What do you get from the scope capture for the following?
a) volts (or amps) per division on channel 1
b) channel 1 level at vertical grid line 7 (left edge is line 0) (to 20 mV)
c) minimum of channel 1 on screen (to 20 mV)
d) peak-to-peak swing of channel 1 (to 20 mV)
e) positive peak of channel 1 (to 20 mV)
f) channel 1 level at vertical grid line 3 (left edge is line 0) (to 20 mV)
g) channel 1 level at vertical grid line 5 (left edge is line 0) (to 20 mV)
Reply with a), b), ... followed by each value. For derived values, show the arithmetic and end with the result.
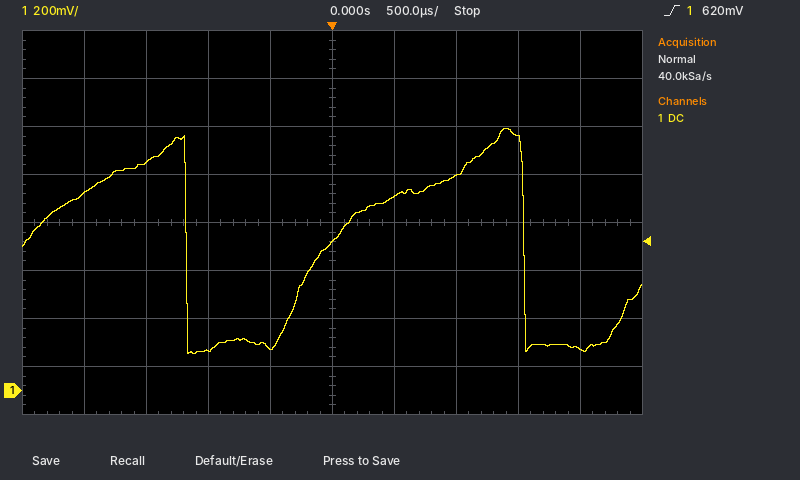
a) 200 mV
b) 900 mV
c) 160 mV
d) 1.10 V − (160 mV) = 940 mV
e) 1.10 V
f) 160 mV
g) 620 mV
